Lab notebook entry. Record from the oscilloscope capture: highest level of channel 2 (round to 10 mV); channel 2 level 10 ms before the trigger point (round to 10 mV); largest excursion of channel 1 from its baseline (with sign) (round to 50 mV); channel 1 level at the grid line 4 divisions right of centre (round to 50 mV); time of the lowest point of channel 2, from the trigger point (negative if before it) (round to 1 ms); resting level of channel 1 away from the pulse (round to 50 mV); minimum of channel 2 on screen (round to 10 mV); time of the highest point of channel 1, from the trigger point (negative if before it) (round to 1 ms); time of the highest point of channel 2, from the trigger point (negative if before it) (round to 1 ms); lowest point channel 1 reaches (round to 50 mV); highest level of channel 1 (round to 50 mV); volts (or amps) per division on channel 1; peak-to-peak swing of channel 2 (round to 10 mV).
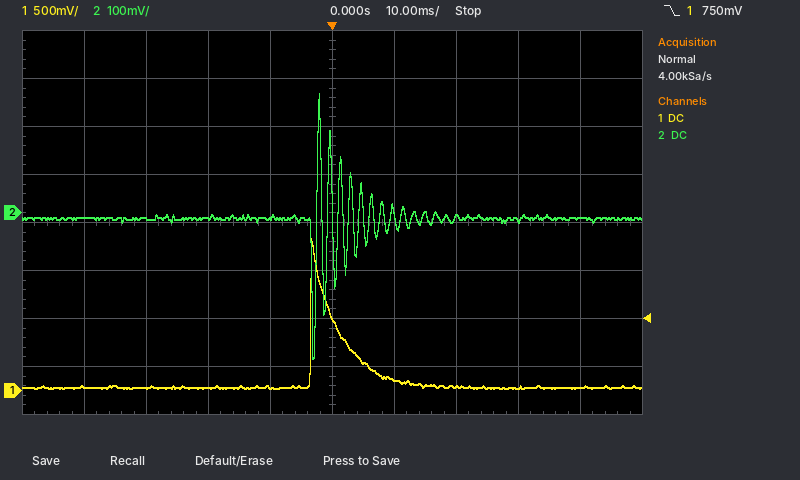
250 mV
-10 mV
+1.55 V
50 mV
-3 ms
50 mV
-300 mV
-3 ms
-2 ms
0 mV
1.60 V
500 mV
550 mV
